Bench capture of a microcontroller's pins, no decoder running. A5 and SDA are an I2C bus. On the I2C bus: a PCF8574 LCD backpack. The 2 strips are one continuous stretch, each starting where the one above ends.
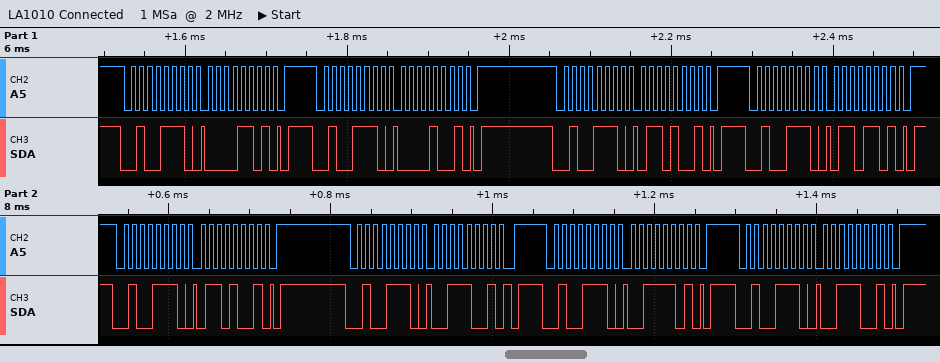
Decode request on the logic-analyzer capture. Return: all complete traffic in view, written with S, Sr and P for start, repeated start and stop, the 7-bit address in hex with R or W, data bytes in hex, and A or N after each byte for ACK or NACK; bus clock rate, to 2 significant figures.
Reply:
S 27W A 0D A P S 27W A 09 A P S 27W A 69 A P S 27W A 6D A P S 27W A 69 A P S 27W A 39 A P S 27W A 3D A P S 27W A 39 A P
100 kHz
